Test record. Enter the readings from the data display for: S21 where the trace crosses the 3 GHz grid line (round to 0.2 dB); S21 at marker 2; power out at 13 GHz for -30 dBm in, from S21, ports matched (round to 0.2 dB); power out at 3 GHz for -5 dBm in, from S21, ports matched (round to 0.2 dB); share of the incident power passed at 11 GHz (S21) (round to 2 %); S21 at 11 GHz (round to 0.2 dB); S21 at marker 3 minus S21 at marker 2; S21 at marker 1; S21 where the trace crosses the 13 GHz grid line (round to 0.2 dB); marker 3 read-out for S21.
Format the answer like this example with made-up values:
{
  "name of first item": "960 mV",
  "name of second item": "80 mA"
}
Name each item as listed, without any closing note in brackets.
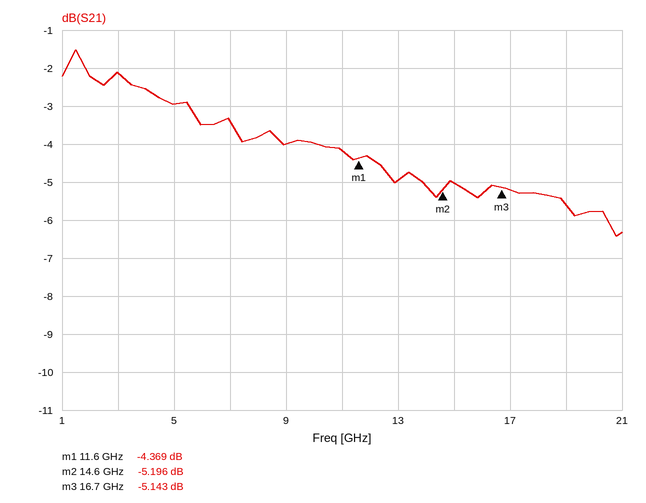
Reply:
{
  "S21 where the trace crosses the 3 GHz grid line": "-2.2 dB",
  "S21 at marker 2": "-5.196 dB",
  "power out at 13 GHz for -30 dBm in, from S21, ports matched": "-35.0 dBm",
  "power out at 3 GHz for -5 dBm in, from S21, ports matched": "-7.2 dBm",
  "share of the incident power passed at 11 GHz (S21)": "38 %",
  "S21 at 11 GHz": "-4.2 dB",
  "S21 at marker 3 minus S21 at marker 2": "0.053 dB",
  "S21 at marker 1": "-4.369 dB",
  "S21 where the trace crosses the 13 GHz grid line": "-5.0 dB",
  "marker 3 read-out for S21": "-5.143 dB"
}
